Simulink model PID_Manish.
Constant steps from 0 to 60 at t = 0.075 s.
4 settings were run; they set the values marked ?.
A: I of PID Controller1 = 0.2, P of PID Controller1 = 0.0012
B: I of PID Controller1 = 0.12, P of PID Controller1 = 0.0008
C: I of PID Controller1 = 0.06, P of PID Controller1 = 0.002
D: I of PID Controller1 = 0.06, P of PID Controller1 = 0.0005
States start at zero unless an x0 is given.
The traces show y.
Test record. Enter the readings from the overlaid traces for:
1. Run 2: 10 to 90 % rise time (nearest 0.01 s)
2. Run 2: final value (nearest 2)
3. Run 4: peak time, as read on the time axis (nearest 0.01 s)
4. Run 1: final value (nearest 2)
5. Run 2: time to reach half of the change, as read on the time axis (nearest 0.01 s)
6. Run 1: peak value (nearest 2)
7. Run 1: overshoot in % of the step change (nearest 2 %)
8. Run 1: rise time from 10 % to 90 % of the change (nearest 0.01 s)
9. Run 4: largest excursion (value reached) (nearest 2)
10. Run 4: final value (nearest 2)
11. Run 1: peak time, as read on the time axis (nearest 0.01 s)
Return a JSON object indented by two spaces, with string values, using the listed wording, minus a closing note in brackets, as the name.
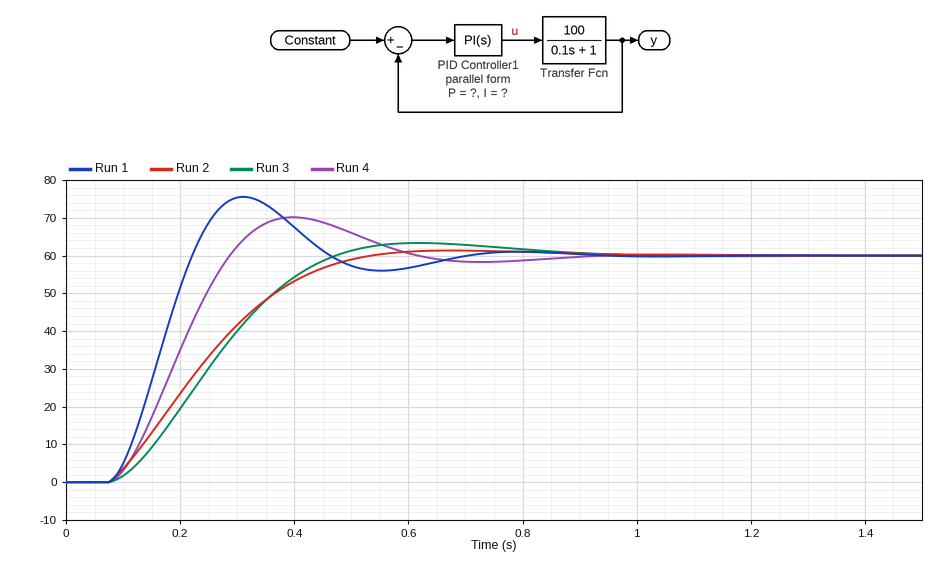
{
  "Run 2: 10 to 90 % rise time": "0.30 s",
  "Run 2: final value": "60",
  "Run 4: peak time, as read on the time axis": "0.40 s",
  "Run 1: final value": "60",
  "Run 2: time to reach half of the change, as read on the time axis": "0.23 s",
  "Run 1: peak value": "76",
  "Run 1: overshoot in % of the step change": "26 %",
  "Run 1: rise time from 10 % to 90 % of the change": "0.10 s",
  "Run 4: largest excursion (value reached)": "70",
  "Run 4: final value": "60",
  "Run 1: peak time, as read on the time axis": "0.31 s"
}
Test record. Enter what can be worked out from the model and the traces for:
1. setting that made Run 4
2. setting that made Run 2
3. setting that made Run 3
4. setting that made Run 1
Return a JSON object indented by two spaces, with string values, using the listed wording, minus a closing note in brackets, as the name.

{
  "setting that made Run 4": "B",
  "setting that made Run 2": "C",
  "setting that made Run 3": "D",
  "setting that made Run 1": "A"
}
